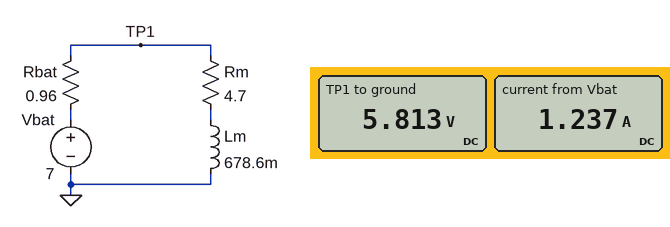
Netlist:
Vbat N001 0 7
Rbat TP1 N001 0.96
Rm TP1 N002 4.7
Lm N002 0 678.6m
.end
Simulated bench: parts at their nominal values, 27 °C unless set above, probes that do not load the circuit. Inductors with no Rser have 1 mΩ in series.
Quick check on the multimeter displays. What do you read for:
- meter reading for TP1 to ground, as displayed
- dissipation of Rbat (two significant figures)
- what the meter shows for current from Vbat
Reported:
5.813 V
1.5 W
1.237 A
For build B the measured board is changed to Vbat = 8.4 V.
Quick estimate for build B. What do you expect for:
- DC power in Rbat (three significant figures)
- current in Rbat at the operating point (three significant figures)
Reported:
2.11 W
1.48 A
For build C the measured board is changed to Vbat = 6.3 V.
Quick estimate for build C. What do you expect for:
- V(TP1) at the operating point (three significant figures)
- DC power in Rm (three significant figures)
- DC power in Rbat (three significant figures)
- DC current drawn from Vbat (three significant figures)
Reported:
5.23 V
5.82 W
1.19 W
1.11 A
